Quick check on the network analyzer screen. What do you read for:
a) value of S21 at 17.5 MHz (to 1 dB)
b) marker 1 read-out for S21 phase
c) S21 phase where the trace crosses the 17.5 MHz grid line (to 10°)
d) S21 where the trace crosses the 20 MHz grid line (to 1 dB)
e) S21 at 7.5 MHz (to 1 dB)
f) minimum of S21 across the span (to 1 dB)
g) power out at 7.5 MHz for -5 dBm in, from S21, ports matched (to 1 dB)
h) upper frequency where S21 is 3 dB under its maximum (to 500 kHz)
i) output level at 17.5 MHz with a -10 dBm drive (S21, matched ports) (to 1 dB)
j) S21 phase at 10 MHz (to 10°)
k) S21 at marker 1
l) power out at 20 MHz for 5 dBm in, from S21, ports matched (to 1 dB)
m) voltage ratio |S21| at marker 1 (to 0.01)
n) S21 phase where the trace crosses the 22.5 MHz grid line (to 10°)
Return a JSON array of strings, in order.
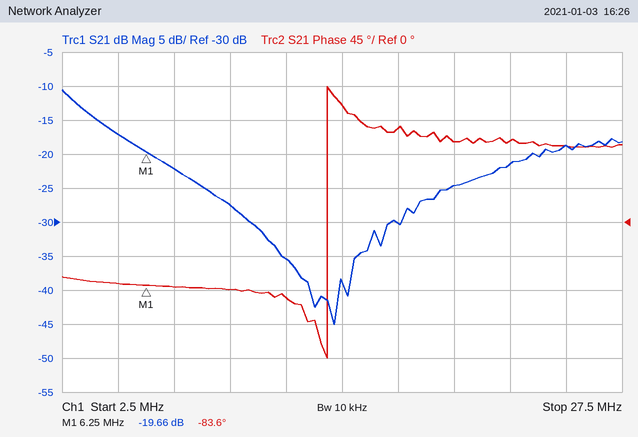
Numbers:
["-30 dB", "-83.6°", "120°", "-25 dB", "-22 dB", "-45 dB", "-27 dBm", "3.5 MHz", "-40 dBm", "-90°", "-19.66 dB", "-20 dBm", "0.10", "110°"]
